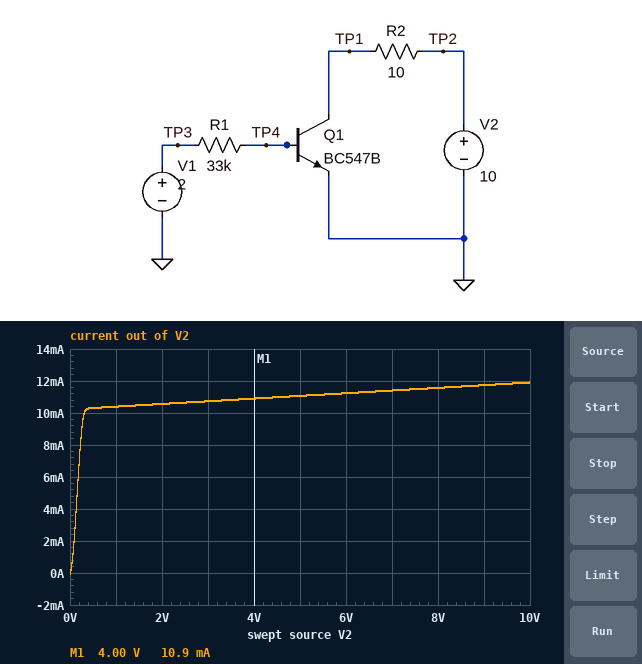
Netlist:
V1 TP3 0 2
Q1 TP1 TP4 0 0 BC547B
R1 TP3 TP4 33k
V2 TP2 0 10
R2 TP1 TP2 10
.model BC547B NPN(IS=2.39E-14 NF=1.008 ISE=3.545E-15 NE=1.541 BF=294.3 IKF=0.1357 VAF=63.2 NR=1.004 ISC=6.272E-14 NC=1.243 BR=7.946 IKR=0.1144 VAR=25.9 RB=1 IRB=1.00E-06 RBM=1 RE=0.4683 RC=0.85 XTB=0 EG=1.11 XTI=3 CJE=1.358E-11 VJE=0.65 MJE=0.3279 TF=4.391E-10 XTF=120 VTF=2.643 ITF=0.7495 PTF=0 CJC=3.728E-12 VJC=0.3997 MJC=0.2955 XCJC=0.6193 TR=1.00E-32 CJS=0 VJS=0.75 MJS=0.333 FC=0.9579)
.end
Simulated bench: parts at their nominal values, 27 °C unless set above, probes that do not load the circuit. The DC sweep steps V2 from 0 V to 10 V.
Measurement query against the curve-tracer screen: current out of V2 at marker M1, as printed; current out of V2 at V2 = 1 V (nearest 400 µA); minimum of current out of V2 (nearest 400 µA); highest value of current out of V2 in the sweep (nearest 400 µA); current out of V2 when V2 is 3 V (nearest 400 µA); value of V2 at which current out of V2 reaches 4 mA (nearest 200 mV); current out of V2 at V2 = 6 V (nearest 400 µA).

10.9 mA
10.4 mA
0 A
12.0 mA
10.8 mA
200 mV
11.2 mA
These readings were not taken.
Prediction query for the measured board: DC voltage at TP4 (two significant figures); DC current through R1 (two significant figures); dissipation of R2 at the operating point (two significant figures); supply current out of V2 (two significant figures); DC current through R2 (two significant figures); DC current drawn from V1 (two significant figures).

710 mV
39 µA
1.4 mW
12 mA
12 mA
39 µA
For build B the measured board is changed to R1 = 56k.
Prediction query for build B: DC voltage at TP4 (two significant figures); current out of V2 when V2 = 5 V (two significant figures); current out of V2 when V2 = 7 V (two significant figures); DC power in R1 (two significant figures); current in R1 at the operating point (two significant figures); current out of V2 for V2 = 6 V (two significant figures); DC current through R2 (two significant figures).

690 mV
6.8 mA
7.0 mA
31 µW
23 µA
6.9 mA
7.3 mA
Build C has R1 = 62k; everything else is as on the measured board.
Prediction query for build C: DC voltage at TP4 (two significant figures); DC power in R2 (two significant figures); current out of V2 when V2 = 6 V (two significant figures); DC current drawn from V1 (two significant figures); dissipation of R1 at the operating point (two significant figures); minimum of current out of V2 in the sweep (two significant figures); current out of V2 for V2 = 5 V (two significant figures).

690 mV
440 µW
6.3 mA
21 µA
28 µW
-32 µA
6.2 mA
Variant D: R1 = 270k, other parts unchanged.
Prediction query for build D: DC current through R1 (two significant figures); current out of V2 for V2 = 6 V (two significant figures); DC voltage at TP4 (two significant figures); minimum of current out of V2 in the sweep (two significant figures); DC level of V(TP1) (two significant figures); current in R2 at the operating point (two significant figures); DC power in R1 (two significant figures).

5.0 µA
1.5 mA
650 mV
-7.6 µA
10 V
1.6 mA
6.8 µW
